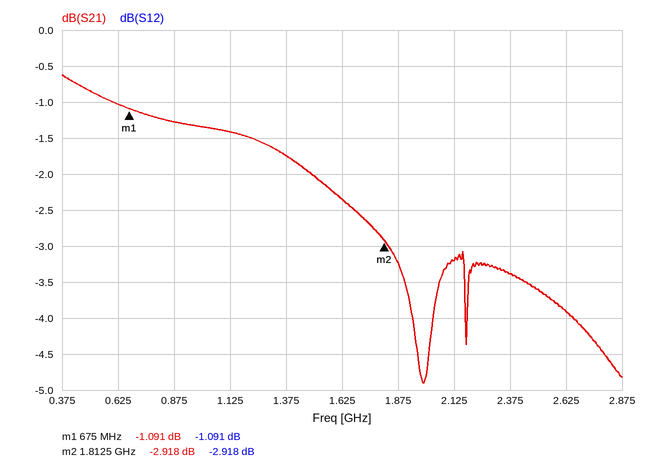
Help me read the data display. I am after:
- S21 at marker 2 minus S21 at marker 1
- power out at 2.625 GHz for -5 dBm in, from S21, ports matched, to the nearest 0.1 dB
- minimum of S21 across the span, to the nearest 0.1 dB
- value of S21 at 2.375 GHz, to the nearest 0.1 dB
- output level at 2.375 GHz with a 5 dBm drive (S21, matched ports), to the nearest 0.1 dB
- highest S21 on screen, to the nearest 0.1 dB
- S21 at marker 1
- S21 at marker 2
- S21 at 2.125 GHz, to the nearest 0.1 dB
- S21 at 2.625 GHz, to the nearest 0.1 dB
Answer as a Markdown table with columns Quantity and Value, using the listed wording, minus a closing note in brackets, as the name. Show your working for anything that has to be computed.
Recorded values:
| Quantity | Value |
|---|---|
| S21 at marker 2 minus S21 at marker 1 | -2.918 − (-1.091) = -1.827 dB |
| power out at 2.625 GHz for -5 dBm in, from S21, ports matched, to the nearest 0.1 dB | -5 dBm + (-3.9 dB) = -8.9 dBm |
| minimum of S21 across the span, to the nearest 0.1 dB | -4.9 dB |
| value of S21 at 2.375 GHz, to the nearest 0.1 dB | -3.4 dB |
| output level at 2.375 GHz with a 5 dBm drive (S21, matched ports), to the nearest 0.1 dB | 5 dBm + (-3.4 dB) = 1.6 dBm |
| highest S21 on screen, to the nearest 0.1 dB | -0.6 dB |
| S21 at marker 1 | -1.091 dB |
| S21 at marker 2 | -2.918 dB |
| S21 at 2.125 GHz, to the nearest 0.1 dB | -3.2 dB |
| S21 at 2.625 GHz, to the nearest 0.1 dB | -3.9 dB |
